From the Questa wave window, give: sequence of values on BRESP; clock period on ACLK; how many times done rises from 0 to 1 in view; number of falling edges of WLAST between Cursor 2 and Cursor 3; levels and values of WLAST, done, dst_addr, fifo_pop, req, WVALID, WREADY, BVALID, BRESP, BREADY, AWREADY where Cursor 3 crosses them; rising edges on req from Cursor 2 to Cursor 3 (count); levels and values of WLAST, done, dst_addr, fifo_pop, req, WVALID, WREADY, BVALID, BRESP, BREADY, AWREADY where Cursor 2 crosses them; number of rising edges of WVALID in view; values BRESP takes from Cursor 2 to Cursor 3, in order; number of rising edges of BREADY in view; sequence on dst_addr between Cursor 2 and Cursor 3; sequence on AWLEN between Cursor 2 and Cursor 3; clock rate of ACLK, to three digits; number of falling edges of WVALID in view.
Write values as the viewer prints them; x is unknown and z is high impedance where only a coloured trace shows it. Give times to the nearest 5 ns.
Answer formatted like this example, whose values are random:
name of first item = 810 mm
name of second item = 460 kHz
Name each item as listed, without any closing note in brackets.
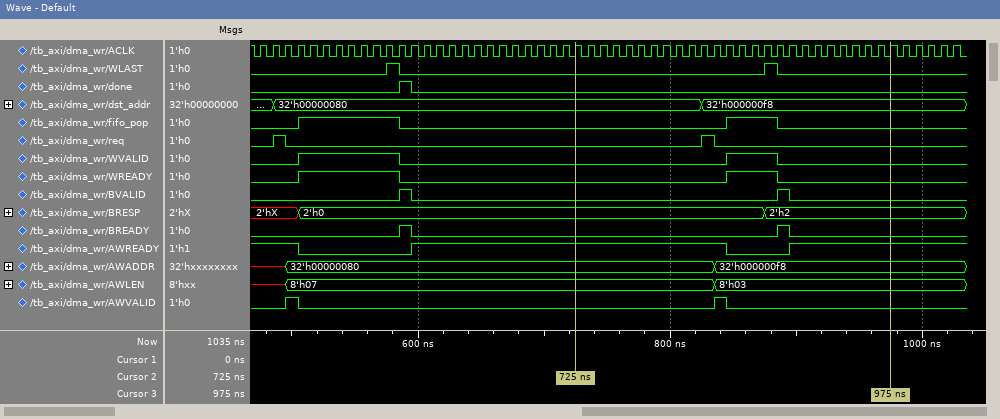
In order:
sequence of values on BRESP = 2'hX, 2'h0, 2'h2
clock period on ACLK = 10 ns
how many times done rises from 0 to 1 in view = 1
number of falling edges of WLAST between Cursor 2 and Cursor 3 = 1
levels and values of WLAST, done, dst_addr, fifo_pop, req, WVALID, WREADY, BVALID, BRESP, BREADY, AWREADY where Cursor 3 crosses them = WLAST=0, done=0, dst_addr=32'h000000f8, fifo_pop=0, req=0, WVALID=0, WREADY=0, BVALID=0, BRESP=2'h2, BREADY=0, AWREADY=1
rising edges on req from Cursor 2 to Cursor 3 = 1
levels and values of WLAST, done, dst_addr, fifo_pop, req, WVALID, WREADY, BVALID, BRESP, BREADY, AWREADY where Cursor 2 crosses them = WLAST=0, done=0, dst_addr=32'h00000080, fifo_pop=0, req=0, WVALID=0, WREADY=0, BVALID=0, BRESP=2'h0, BREADY=0, AWREADY=1
number of rising edges of WVALID in view = 2
values BRESP takes from Cursor 2 to Cursor 3, in order = 2'h0, 2'h2
number of rising edges of BREADY in view = 2
sequence on dst_addr between Cursor 2 and Cursor 3 = 32'h00000080, 32'h000000f8
sequence on AWLEN between Cursor 2 and Cursor 3 = 8'h07, 8'h03
clock rate of ACLK, to three digits = 100 MHz
number of falling edges of WVALID in view = 2
